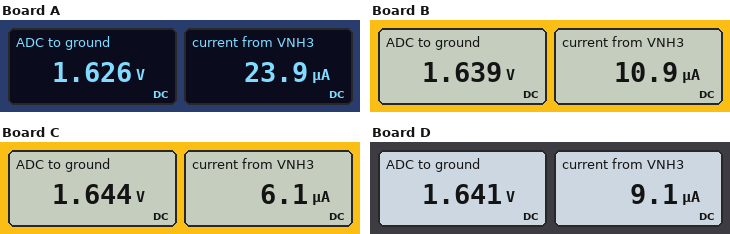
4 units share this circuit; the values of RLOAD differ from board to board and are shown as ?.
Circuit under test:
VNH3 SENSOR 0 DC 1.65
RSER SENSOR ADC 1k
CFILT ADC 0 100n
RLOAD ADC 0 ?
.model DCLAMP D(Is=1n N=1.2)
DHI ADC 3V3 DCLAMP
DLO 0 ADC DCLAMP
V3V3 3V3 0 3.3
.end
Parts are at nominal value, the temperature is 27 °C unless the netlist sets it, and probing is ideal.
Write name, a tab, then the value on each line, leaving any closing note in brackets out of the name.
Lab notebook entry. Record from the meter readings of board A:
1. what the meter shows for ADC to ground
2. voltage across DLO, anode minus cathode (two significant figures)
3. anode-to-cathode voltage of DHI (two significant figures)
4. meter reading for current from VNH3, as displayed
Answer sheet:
what the meter shows for ADC to ground	1.626 V
voltage across DLO, anode minus cathode	-1.6 V
anode-to-cathode voltage of DHI	-1.7 V
meter reading for current from VNH3, as displayed	23.9 µA
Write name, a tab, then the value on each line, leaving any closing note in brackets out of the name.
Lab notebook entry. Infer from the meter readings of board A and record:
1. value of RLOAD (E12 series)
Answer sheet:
value of RLOAD	68 kΩ
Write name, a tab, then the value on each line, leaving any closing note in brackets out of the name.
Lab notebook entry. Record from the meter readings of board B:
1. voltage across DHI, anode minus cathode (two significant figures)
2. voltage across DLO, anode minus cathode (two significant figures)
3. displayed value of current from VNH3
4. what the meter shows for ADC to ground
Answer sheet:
voltage across DHI, anode minus cathode	-1.7 V
voltage across DLO, anode minus cathode	-1.6 V
displayed value of current from VNH3	10.9 µA
what the meter shows for ADC to ground	1.639 V
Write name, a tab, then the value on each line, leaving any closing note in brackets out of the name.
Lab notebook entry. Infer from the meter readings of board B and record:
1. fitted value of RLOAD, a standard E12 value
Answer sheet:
fitted value of RLOAD, a standard E12 value	150 kΩ
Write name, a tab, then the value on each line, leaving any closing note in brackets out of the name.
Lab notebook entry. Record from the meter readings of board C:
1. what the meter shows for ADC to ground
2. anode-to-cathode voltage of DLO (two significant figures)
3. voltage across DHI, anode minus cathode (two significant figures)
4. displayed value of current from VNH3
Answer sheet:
what the meter shows for ADC to ground	1.644 V
anode-to-cathode voltage of DLO	-1.6 V
voltage across DHI, anode minus cathode	-1.7 V
displayed value of current from VNH3	6.1 µA
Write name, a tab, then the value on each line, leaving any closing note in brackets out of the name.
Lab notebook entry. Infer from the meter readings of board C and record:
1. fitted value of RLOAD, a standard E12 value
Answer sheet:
fitted value of RLOAD, a standard E12 value	270 kΩ
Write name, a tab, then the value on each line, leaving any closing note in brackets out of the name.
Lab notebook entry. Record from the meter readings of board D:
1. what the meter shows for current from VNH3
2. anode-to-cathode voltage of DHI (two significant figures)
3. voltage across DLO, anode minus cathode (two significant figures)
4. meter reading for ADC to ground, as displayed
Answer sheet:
what the meter shows for current from VNH3	9.1 µA
anode-to-cathode voltage of DHI	-1.7 V
voltage across DLO, anode minus cathode	-1.6 V
meter reading for ADC to ground, as displayed	1.641 V
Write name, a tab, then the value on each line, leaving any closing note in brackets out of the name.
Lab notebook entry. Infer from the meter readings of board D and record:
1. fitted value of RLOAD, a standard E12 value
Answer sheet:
fitted value of RLOAD, a standard E12 value	180 kΩ
